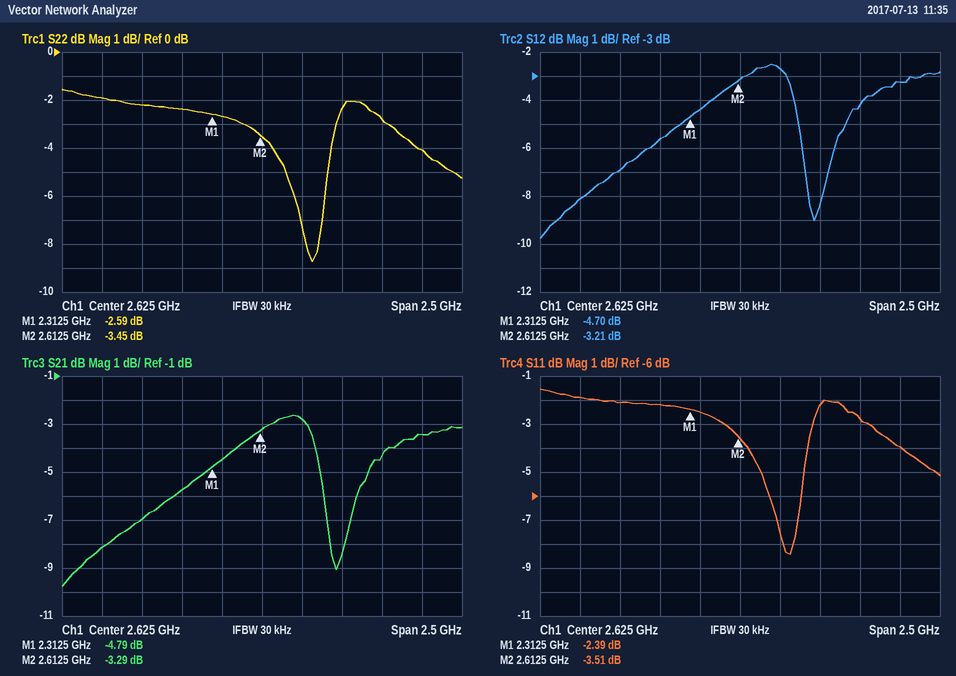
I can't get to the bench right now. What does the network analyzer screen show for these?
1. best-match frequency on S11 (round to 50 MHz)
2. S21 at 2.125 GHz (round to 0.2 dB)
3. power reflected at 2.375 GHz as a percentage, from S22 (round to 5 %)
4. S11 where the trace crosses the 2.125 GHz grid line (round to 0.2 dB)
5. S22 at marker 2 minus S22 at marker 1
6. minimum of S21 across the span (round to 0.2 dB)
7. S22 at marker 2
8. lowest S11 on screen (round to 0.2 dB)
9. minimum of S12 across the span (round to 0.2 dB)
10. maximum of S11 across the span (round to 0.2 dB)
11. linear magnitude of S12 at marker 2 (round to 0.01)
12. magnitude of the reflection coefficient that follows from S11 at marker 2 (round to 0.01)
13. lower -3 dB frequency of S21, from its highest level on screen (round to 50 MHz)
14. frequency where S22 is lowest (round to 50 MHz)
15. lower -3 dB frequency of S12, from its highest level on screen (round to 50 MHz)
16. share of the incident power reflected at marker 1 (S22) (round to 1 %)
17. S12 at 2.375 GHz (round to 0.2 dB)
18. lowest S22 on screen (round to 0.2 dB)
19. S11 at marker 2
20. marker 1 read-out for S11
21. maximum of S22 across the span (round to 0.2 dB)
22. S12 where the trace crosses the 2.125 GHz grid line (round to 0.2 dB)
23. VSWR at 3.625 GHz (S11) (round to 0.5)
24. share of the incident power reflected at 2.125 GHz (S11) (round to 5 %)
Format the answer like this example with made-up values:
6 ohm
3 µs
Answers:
2.95 GHz
-5.8 dB
55 %
-2.2 dB
-0.86 dB
-9.8 dB
-3.45 dB
-8.4 dB
-9.8 dB
-1.6 dB
0.69
0.67
2.15 GHz
2.95 GHz
2.15 GHz
55 %
-4.4 dB
-8.8 dB
-3.51 dB
-2.39 dB
-1.6 dB
-5.6 dB
4.5
60 %
